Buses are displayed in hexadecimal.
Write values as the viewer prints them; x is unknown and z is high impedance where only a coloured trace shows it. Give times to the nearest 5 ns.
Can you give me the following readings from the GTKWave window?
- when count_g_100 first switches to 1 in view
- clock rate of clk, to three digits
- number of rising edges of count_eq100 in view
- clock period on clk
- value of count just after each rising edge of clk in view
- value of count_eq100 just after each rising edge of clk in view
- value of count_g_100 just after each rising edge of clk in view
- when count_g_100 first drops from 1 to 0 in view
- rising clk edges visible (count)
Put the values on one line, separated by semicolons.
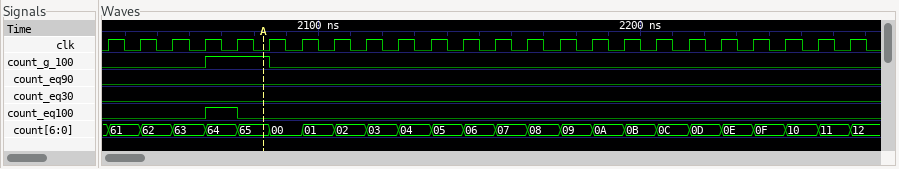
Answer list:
2065 ns; 100 MHz; 1; 10 ns; 61, 62, 63, 64, 65, 00, 01, 02, 03, 04, 05, 06, 07, 08, 09, 0A, 0B, 0C, 0D, 0E, 0F, 10, 11, 12; 0 0 0 1 0 0 0 0 0 0 0 0 0 0 0 0 0 0 0 0 0 0 0 0; 0 0 0 1 1 0 0 0 0 0 0 0 0 0 0 0 0 0 0 0 0 0 0 0; 2085 ns; 24
